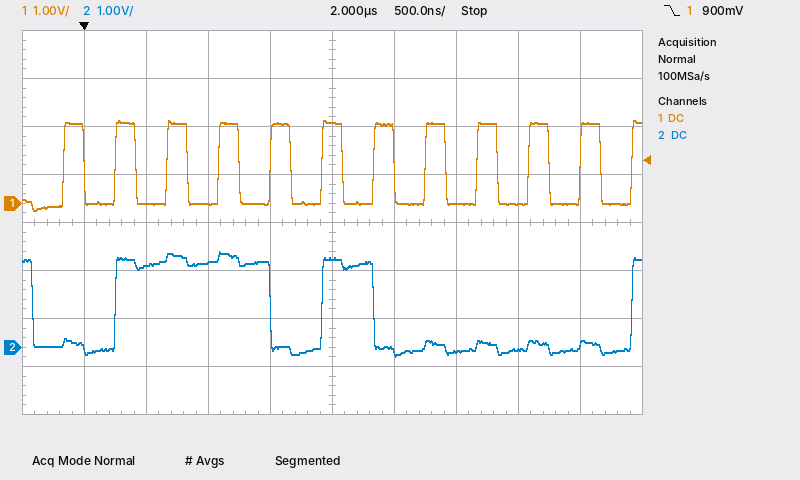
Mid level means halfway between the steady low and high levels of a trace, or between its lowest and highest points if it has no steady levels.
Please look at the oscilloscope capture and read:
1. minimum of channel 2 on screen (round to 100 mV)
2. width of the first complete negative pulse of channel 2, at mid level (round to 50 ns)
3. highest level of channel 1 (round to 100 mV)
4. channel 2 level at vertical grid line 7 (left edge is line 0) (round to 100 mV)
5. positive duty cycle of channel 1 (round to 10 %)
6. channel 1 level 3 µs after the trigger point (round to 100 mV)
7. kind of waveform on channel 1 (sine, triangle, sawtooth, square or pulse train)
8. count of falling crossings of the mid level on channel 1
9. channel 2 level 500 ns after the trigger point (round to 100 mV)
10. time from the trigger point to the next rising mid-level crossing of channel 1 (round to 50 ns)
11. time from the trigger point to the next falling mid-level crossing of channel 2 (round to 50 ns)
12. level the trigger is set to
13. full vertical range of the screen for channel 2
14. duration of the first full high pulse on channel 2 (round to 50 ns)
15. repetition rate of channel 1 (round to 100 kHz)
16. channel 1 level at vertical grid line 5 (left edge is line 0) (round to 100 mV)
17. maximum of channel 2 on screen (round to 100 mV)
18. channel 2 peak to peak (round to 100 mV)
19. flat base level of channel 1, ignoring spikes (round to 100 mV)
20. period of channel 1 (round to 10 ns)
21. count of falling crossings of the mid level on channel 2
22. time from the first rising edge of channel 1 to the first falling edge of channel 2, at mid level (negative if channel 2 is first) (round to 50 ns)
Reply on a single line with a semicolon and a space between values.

-200 mV; 650 ns; 1.7 V; -100 mV; 40 %; 0.0 V; pulse train; 11; 1.7 V; 250 ns; 1.50 µs; 900 mV; 8 V; 1.25 µs; 2.4 MHz; 1.7 V; 2.0 V; 2.2 V; 0.0 V; 420 ns; 3; -250 ns
